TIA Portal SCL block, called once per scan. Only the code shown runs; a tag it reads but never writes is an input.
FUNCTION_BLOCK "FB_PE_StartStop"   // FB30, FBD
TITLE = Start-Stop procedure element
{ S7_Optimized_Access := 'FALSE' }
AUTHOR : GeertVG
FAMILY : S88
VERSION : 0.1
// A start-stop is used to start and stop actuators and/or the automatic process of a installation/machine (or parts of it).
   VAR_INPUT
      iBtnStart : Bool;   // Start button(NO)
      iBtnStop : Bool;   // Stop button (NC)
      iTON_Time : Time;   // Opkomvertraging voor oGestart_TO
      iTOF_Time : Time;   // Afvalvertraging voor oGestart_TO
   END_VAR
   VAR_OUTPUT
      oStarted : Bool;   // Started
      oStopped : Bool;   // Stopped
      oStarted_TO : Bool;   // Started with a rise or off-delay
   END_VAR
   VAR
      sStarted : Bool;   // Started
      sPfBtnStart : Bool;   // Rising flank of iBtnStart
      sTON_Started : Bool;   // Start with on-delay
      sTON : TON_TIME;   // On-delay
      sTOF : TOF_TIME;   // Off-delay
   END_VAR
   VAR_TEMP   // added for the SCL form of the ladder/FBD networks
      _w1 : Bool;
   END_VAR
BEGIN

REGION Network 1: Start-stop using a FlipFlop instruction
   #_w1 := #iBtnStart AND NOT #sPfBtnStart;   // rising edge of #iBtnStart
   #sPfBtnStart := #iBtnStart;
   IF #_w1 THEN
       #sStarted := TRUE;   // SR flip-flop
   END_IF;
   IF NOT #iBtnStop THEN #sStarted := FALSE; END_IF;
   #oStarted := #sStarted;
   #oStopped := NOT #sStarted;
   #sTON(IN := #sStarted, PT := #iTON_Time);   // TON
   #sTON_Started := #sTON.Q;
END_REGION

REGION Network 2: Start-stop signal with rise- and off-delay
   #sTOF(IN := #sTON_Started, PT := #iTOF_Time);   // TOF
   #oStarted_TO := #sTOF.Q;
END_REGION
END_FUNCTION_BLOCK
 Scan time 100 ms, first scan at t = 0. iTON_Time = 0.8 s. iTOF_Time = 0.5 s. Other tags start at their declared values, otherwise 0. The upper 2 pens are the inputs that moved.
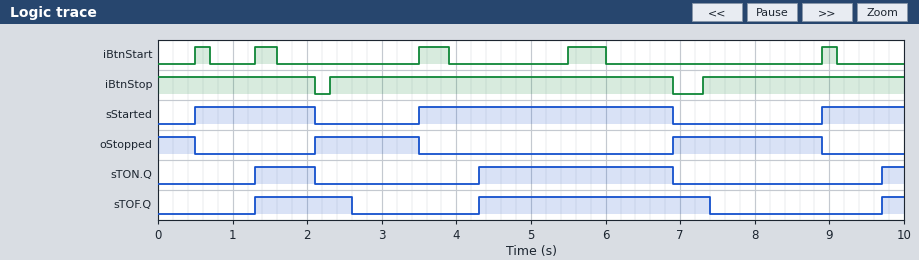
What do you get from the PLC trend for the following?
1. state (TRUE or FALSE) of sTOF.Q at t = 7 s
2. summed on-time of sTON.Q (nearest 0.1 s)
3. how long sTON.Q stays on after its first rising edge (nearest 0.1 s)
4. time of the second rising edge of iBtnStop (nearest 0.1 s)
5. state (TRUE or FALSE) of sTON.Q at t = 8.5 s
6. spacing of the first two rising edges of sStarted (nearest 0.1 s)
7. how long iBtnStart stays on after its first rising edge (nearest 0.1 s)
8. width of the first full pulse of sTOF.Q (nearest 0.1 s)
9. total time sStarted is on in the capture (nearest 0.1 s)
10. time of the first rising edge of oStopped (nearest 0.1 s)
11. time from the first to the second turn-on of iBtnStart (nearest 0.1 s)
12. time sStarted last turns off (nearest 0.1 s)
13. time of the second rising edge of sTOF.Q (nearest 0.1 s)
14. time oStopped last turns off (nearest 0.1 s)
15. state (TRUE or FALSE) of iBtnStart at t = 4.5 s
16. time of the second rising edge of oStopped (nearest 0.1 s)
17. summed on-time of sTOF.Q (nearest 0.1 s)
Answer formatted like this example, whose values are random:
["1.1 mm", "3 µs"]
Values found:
["TRUE", "3.7 s", "0.8 s", "7.3 s", "FALSE", "3.0 s", "0.2 s", "1.3 s", "6.1 s", "2.1 s", "0.8 s", "6.9 s", "4.3 s", "8.9 s", "FALSE", "6.9 s", "4.7 s"]
